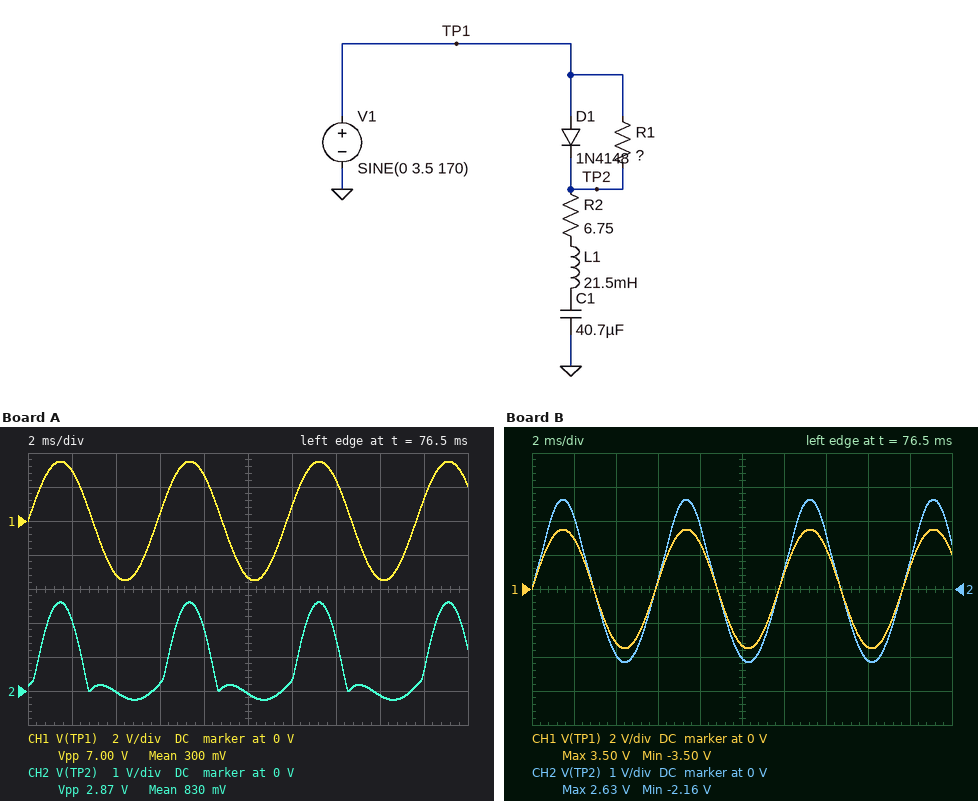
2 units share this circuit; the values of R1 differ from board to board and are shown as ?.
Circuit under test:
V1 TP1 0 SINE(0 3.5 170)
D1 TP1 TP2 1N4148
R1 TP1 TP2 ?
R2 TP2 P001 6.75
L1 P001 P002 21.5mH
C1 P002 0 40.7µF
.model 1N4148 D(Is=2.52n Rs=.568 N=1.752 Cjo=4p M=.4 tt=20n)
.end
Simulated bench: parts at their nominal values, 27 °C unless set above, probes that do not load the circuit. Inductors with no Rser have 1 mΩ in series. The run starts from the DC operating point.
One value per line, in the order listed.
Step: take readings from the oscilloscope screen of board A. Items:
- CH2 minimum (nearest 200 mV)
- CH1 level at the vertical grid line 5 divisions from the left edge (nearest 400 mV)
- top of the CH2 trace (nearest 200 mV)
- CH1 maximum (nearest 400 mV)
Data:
-200 mV
-3.2 V
2.6 V
3.6 V
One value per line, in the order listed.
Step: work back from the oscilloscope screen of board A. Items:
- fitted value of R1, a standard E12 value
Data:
18 Ω
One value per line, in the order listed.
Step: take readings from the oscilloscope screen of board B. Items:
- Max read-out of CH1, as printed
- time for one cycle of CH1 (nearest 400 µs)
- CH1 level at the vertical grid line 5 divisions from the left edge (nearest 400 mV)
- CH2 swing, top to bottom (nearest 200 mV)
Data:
3.50 V
6.0 ms
-3.2 V
4.8 V
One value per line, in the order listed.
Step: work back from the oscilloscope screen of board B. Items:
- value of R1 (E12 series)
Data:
3.9 Ω
